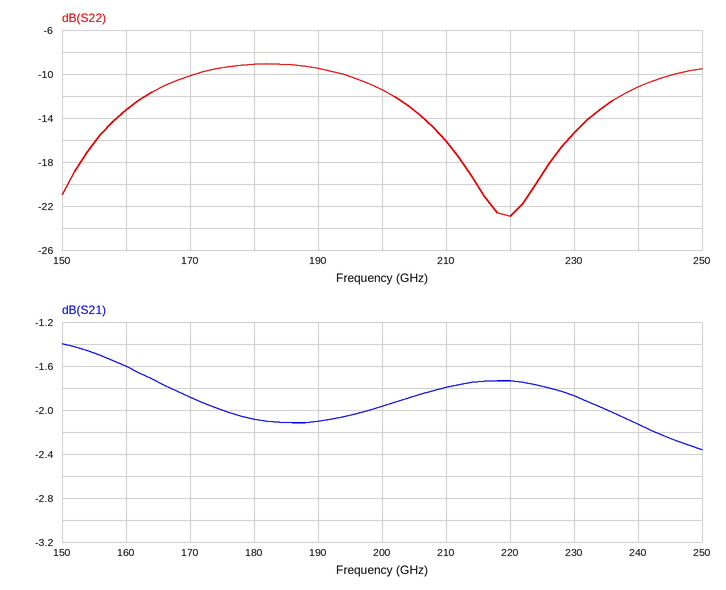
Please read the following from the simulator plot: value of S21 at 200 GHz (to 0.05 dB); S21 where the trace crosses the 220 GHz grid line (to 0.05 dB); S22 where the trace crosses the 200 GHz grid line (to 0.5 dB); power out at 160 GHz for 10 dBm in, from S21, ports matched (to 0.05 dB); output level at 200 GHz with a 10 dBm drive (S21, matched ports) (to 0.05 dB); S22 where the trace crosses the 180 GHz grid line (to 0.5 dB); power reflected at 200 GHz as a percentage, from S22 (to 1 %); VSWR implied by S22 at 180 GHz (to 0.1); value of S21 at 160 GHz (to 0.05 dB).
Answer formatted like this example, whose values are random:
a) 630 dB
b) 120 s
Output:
a) -1.95 dB
b) -1.75 dB
c) -11.5 dB
d) 8.40 dBm
e) 8.05 dBm
f) -9.0 dB
g) 7 %
h) 2.1
i) -1.60 dB
